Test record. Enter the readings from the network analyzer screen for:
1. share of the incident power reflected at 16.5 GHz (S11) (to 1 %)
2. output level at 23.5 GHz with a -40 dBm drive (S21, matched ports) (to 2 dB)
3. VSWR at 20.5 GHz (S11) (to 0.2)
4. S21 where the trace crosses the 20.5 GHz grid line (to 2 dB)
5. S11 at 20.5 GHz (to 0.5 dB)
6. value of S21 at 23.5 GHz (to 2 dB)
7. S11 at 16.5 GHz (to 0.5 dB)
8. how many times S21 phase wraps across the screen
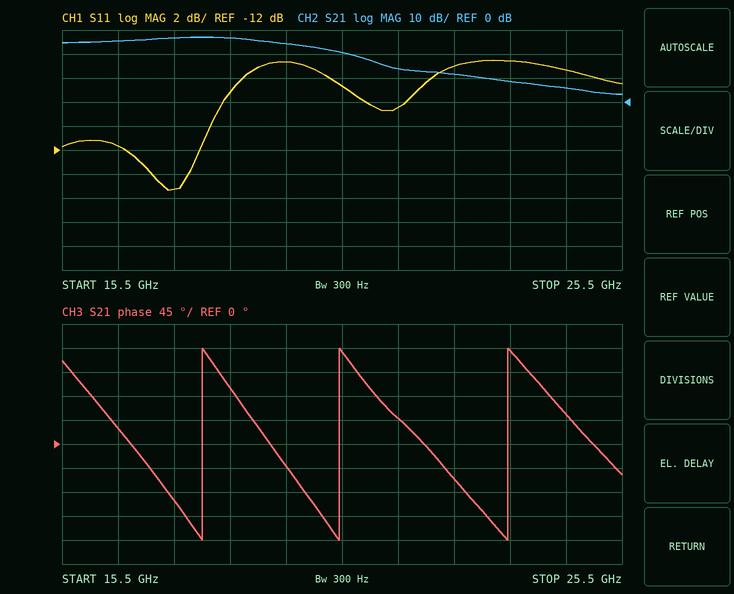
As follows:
7 %
-32 dBm
2.8
20 dB
-6.5 dB
8 dB
-11.5 dB
3
